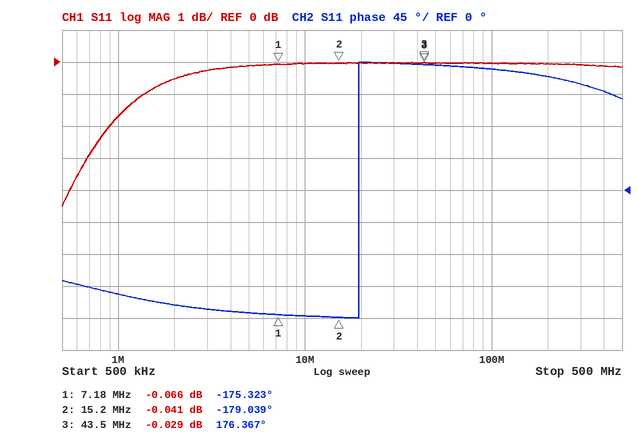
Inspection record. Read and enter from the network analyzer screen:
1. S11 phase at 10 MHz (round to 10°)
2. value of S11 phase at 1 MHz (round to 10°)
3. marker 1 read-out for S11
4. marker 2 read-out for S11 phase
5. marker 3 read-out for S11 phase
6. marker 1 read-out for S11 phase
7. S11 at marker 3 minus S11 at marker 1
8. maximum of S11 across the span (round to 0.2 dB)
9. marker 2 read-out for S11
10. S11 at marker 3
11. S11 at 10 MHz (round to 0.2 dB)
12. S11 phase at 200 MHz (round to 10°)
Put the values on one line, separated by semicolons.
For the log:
-180°; -150°; -0.066 dB; -179.039°; 176.367°; -175.323°; 0.037 dB; 0.0 dB; -0.041 dB; -0.029 dB; 0.0 dB; 160°
